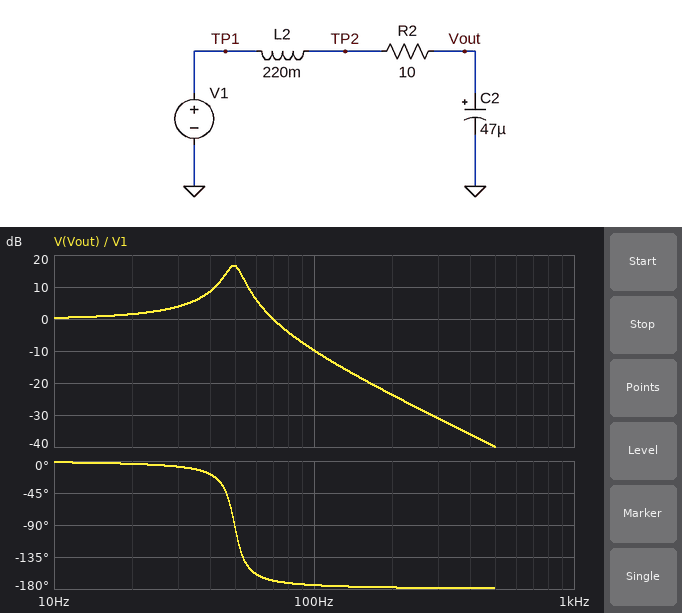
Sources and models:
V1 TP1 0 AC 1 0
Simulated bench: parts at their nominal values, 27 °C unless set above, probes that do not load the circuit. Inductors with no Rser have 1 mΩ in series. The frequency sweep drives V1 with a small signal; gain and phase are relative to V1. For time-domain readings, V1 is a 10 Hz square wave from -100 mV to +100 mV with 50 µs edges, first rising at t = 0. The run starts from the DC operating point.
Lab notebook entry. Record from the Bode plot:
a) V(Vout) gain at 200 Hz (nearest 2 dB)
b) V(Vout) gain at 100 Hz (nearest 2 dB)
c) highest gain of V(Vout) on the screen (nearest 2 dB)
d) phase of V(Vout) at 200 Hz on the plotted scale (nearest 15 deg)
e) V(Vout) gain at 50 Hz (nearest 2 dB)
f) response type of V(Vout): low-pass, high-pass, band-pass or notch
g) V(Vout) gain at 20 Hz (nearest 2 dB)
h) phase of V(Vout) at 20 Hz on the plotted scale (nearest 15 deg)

-24 dB
-10 dB
16 dB
-180 deg
16 dB
low-pass
2 dB
0 deg
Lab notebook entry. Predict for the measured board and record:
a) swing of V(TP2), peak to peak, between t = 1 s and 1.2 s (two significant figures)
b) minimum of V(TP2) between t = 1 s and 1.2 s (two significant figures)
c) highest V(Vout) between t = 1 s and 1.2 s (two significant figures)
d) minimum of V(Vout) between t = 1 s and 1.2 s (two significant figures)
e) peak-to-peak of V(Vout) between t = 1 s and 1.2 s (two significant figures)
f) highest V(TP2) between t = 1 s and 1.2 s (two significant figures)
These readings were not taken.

660 mV
-330 mV
330 mV
-330 mV
660 mV
330 mV
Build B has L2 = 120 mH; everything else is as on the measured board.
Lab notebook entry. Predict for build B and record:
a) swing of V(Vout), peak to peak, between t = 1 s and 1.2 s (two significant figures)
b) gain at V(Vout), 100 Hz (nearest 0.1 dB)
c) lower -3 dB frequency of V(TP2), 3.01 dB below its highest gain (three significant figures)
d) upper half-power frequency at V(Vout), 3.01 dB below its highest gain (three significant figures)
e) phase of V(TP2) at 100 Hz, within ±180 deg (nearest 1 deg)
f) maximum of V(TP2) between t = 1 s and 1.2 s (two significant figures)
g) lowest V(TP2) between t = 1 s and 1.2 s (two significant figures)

510 mV
-2.0 dB
59.4 Hz
72.7 Hz
-150 deg
260 mV
-260 mV
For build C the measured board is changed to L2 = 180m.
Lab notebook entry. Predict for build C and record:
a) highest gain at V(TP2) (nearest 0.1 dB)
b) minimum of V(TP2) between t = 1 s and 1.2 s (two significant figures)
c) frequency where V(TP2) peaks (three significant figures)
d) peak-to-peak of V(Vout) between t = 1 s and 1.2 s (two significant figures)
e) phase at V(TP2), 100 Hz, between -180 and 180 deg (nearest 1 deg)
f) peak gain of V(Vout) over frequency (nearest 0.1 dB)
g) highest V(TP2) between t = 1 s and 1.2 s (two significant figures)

16.0 dB
-260 mV
54.4 Hz
520 mV
-156 deg
15.9 dB
260 mV
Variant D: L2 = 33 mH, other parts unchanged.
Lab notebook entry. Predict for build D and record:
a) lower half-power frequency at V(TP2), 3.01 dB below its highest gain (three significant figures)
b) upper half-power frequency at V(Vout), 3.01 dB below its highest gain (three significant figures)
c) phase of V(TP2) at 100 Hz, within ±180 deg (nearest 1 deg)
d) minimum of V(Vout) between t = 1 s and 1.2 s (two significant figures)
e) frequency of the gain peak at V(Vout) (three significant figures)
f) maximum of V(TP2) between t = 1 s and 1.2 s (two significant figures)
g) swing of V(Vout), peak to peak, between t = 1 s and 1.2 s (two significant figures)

96.9 Hz
146 Hz
-21 deg
-210 mV
123 Hz
220 mV
420 mV
